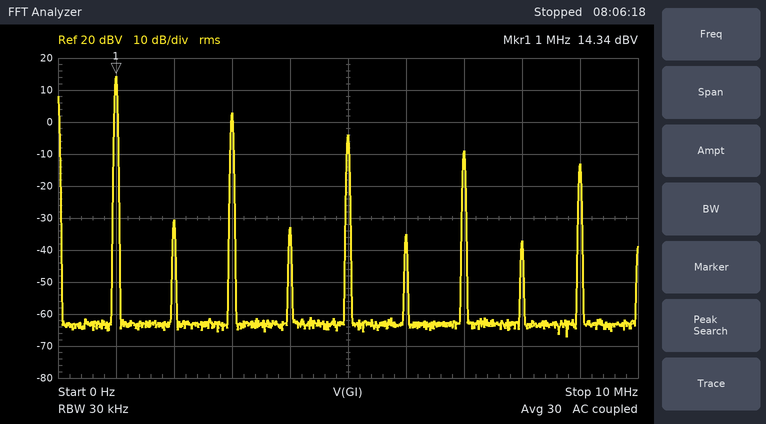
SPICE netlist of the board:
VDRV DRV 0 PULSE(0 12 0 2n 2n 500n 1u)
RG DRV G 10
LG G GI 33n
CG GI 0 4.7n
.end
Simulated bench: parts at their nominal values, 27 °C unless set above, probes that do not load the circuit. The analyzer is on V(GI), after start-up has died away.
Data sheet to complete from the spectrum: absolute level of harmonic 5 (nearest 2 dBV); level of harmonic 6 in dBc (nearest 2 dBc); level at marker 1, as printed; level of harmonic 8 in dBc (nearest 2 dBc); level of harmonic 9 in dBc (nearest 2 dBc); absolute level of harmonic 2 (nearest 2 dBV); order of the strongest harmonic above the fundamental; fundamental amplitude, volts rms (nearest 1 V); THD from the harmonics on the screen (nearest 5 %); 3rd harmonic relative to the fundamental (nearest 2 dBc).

-4 dBV
-50 dBc
14.34 dBV
-52 dBc
-28 dBc
-30 dBV
3
5 V
30 %
-12 dBc
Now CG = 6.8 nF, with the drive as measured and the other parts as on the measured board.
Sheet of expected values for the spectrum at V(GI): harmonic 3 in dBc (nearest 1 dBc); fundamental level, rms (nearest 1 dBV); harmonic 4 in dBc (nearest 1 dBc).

-13 dBc
14 dBV
-49 dBc
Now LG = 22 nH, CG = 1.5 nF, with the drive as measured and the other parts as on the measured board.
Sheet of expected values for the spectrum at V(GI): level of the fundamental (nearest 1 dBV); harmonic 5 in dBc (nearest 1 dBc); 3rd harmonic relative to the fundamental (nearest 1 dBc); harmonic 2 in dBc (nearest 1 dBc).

15 dBV
-15 dBc
-10 dBc
-44 dBc
